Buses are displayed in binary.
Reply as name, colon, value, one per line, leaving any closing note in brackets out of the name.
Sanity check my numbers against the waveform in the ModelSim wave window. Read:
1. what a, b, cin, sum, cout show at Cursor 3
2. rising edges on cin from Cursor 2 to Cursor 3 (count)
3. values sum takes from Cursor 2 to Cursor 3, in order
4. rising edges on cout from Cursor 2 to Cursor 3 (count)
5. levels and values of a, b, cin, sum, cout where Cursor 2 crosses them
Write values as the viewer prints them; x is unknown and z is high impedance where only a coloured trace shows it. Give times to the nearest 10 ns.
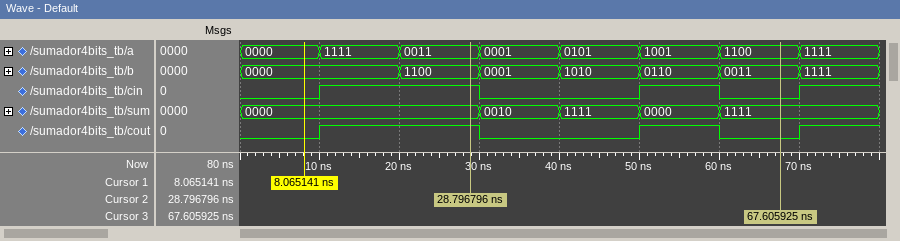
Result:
what a, b, cin, sum, cout show at Cursor 3: a=1100, b=0011, cin=0, sum=1111, cout=0
rising edges on cin from Cursor 2 to Cursor 3: 1
values sum takes from Cursor 2 to Cursor 3, in order: 0000, 0010, 1111, 0000, 1111
rising edges on cout from Cursor 2 to Cursor 3: 1
levels and values of a, b, cin, sum, cout where Cursor 2 crosses them: a=0011, b=1100, cin=1, sum=0000, cout=1
